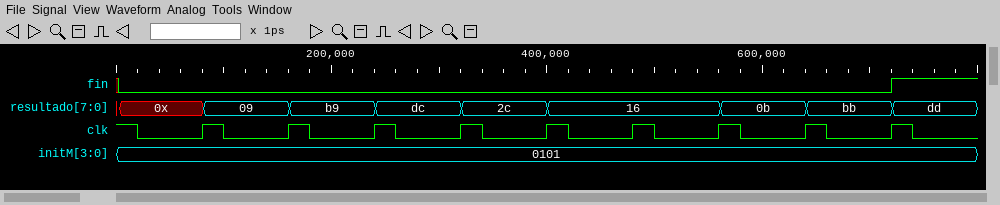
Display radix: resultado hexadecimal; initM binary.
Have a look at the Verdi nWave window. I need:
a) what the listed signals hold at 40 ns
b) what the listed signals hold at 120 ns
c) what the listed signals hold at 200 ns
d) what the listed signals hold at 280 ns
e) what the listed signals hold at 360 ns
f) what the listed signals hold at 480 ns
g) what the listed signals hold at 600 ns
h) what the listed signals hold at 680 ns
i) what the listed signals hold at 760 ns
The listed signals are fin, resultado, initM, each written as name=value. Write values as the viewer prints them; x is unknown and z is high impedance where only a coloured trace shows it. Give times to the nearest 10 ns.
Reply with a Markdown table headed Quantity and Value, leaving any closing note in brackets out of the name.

| Quantity | Value |
|---|---|
| what the listed signals hold at 40 ns | fin=0, resultado=0x, initM=0101 |
| what the listed signals hold at 120 ns | fin=0, resultado=09, initM=0101 |
| what the listed signals hold at 200 ns | fin=0, resultado=b9, initM=0101 |
| what the listed signals hold at 280 ns | fin=0, resultado=dc, initM=0101 |
| what the listed signals hold at 360 ns | fin=0, resultado=2c, initM=0101 |
| what the listed signals hold at 480 ns | fin=0, resultado=16, initM=0101 |
| what the listed signals hold at 600 ns | fin=0, resultado=0b, initM=0101 |
| what the listed signals hold at 680 ns | fin=0, resultado=bb, initM=0101 |
| what the listed signals hold at 760 ns | fin=1, resultado=dd, initM=0101 |
